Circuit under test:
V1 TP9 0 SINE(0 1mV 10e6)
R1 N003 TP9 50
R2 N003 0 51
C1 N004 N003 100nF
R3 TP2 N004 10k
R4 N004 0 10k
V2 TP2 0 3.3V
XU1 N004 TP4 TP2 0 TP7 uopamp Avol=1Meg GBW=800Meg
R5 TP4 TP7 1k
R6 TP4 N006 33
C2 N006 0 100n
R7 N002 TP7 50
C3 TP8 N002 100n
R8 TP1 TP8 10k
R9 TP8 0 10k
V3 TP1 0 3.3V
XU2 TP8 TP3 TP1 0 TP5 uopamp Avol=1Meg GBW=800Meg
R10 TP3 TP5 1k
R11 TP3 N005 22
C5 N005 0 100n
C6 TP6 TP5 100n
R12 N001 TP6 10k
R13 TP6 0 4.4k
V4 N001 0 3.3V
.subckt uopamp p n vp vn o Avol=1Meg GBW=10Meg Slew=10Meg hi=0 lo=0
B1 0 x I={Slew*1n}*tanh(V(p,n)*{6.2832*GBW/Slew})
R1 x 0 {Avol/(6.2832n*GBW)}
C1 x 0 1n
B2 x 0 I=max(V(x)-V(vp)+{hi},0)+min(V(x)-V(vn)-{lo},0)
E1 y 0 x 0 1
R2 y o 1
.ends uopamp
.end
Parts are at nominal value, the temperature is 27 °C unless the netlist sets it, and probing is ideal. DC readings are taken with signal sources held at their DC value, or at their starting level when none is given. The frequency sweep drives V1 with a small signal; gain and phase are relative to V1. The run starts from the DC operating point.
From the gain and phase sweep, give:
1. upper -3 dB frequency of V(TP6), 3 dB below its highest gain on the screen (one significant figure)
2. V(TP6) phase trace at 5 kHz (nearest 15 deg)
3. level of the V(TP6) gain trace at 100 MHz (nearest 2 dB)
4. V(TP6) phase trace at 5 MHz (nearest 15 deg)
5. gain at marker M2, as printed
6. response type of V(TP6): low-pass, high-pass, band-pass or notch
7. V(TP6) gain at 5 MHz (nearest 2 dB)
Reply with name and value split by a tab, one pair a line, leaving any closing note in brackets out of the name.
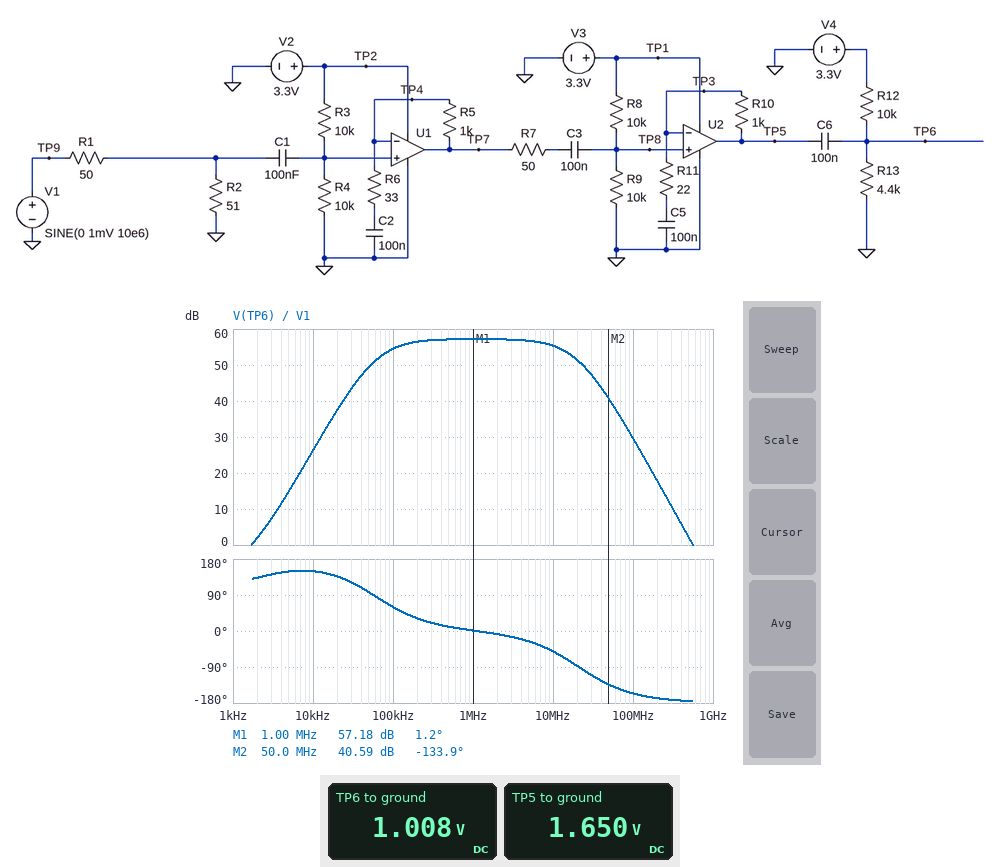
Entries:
upper -3 dB frequency of V(TP6), 3 dB below its highest gain on the screen	10 MHz
V(TP6) phase trace at 5 kHz	150 deg
level of the V(TP6) gain trace at 100 MHz	30 dB
V(TP6) phase trace at 5 MHz	-30 deg
gain at marker M2, as printed	40.59 dB
response type of V(TP6): low-pass, high-pass, band-pass or notch	band-pass
V(TP6) gain at 5 MHz	56 dB
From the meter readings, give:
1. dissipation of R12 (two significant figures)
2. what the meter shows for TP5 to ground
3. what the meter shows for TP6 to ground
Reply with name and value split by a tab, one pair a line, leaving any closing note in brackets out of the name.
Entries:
dissipation of R12	530 µW
what the meter shows for TP5 to ground	1.650 V
what the meter shows for TP6 to ground	1.008 V
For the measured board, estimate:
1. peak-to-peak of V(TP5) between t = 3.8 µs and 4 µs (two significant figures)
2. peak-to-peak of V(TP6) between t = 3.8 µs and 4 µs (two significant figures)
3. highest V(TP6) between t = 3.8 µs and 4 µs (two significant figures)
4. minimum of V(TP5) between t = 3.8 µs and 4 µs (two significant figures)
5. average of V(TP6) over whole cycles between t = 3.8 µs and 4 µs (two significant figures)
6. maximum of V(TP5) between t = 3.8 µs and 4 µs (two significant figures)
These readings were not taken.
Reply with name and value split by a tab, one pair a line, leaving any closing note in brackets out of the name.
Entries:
peak-to-peak of V(TP5) between t = 3.8 µs and 4 µs	470 mV
peak-to-peak of V(TP6) between t = 3.8 µs and 4 µs	470 mV
highest V(TP6) between t = 3.8 µs and 4 µs	1.2 V
minimum of V(TP5) between t = 3.8 µs and 4 µs	1.4 V
average of V(TP6) over whole cycles between t = 3.8 µs and 4 µs	1.0 V
maximum of V(TP5) between t = 3.8 µs and 4 µs	1.9 V
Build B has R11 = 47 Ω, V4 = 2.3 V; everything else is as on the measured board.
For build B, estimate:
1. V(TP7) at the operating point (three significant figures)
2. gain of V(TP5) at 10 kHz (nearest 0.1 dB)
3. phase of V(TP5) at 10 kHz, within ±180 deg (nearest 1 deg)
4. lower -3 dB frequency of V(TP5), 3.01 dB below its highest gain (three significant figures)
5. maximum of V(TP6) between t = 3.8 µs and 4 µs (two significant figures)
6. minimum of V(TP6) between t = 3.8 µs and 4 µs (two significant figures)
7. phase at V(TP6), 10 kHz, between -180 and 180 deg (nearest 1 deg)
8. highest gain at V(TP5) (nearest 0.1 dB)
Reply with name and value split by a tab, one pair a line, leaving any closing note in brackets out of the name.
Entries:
V(TP7) at the operating point	1.65 V
gain of V(TP5) at 10 kHz	26.2 dB
phase of V(TP5) at 10 kHz, within ±180 deg	138 deg
lower -3 dB frequency of V(TP5), 3.01 dB below its highest gain	63.9 kHz
maximum of V(TP6) between t = 3.8 µs and 4 µs	930 mV
minimum of V(TP6) between t = 3.8 µs and 4 µs	470 mV
phase at V(TP6), 10 kHz, between -180 and 180 deg	141 deg
highest gain at V(TP5)	50.8 dB
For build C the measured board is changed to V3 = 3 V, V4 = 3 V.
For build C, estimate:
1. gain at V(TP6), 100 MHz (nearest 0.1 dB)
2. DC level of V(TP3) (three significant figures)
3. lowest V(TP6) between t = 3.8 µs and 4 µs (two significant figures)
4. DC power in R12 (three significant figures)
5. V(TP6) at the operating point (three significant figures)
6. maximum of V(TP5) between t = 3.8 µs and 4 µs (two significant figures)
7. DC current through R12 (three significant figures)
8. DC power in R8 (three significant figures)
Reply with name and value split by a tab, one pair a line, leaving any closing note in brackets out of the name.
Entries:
gain at V(TP6), 100 MHz	29.6 dB
DC level of V(TP3)	1.50 V
lowest V(TP6) between t = 3.8 µs and 4 µs	680 mV
DC power in R12	434 µW
V(TP6) at the operating point	917 mV
maximum of V(TP5) between t = 3.8 µs and 4 µs	1.7 V
DC current through R12	208 µA
DC power in R8	225 µW
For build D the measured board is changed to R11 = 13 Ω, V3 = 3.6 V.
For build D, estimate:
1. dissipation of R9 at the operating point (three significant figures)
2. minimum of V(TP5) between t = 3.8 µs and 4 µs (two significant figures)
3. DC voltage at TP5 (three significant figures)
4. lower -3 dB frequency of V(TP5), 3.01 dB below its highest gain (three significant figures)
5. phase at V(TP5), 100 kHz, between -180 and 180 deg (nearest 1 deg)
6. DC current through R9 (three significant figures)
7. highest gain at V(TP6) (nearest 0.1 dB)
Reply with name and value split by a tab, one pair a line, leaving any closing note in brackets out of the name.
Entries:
dissipation of R9 at the operating point	324 µW
minimum of V(TP5) between t = 3.8 µs and 4 µs	1.6 V
DC voltage at TP5	1.80 V
lower -3 dB frequency of V(TP5), 3.01 dB below its highest gain	136 kHz
phase at V(TP5), 100 kHz, between -180 and 180 deg	75 deg
DC current through R9	180 µA
highest gain at V(TP6)	61.7 dB
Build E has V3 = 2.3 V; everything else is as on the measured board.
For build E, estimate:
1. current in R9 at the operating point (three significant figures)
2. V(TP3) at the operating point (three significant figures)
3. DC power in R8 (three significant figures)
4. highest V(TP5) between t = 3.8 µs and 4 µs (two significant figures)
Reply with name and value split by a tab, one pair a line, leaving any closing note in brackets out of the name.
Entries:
current in R9 at the operating point	115 µA
V(TP3) at the operating point	1.15 V
DC power in R8	132 µW
highest V(TP5) between t = 3.8 µs and 4 µs	1.4 V
